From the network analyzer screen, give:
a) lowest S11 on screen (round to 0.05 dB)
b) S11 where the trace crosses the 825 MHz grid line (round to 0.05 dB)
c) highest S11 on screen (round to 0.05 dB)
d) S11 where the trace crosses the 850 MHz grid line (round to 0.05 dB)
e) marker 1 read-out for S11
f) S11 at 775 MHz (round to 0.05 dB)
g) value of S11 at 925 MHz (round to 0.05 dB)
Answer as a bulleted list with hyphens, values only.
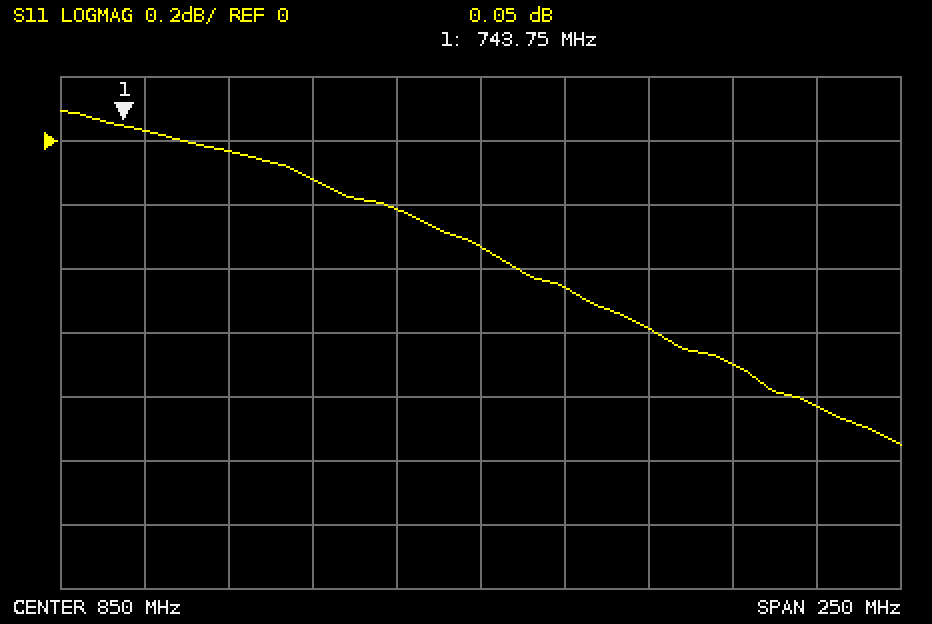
- -0.95 dB
- -0.20 dB
- 0.10 dB
- -0.35 dB
- 0.05 dB
- -0.05 dB
- -0.70 dB
